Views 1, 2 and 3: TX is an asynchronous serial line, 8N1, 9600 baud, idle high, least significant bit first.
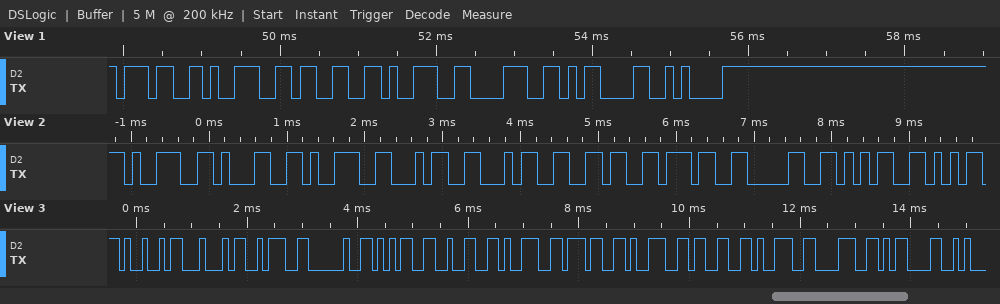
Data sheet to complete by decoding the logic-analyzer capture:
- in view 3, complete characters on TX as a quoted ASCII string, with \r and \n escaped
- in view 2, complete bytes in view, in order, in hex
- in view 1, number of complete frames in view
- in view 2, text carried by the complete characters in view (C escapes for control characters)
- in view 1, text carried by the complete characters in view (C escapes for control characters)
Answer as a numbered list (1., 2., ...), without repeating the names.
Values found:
1. "ID: 52979398\r"
2. 39 31 39 34 34 36 37 30 35
3. 7
4. "919446705"
5. "79398\r\n"
